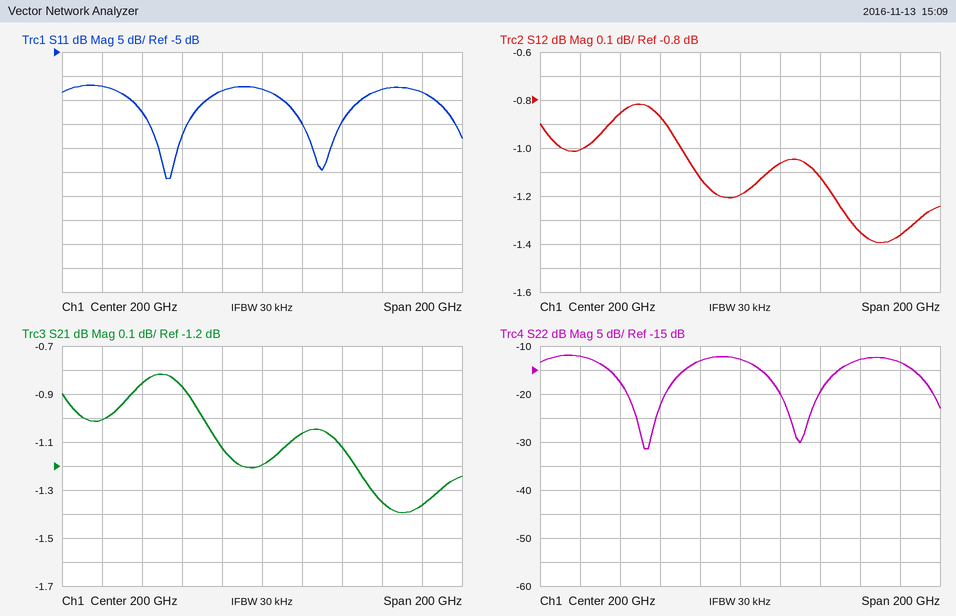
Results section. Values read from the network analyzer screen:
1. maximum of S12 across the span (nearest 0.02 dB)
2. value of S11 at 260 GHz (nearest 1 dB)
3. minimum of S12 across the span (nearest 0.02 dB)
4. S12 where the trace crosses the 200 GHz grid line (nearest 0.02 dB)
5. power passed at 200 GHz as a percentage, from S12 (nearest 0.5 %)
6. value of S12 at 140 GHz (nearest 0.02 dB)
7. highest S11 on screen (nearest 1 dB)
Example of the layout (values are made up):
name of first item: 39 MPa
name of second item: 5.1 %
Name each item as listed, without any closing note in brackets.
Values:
maximum of S12 across the span: -0.82 dB
value of S11 at 260 GHz: -13 dB
minimum of S12 across the span: -1.40 dB
S12 where the trace crosses the 200 GHz grid line: -1.20 dB
power passed at 200 GHz as a percentage, from S12: 76.0 %
value of S12 at 140 GHz: -0.86 dB
highest S11 on screen: -12 dB
